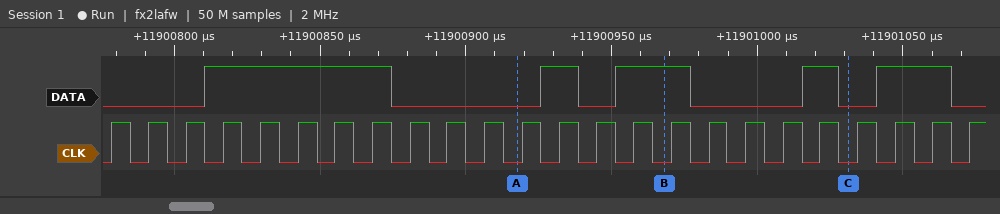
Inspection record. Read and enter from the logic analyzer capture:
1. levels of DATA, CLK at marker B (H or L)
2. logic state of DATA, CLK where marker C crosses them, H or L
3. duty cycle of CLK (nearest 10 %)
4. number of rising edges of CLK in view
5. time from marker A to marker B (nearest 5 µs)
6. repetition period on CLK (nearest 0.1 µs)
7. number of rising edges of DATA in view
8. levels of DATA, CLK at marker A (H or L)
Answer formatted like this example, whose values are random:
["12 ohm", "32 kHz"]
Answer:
["DATA=H, CLK=L", "DATA=L, CLK=L", "50 %", "24", "50 µs", "12.8 µs", "5", "DATA=L, CLK=L"]
